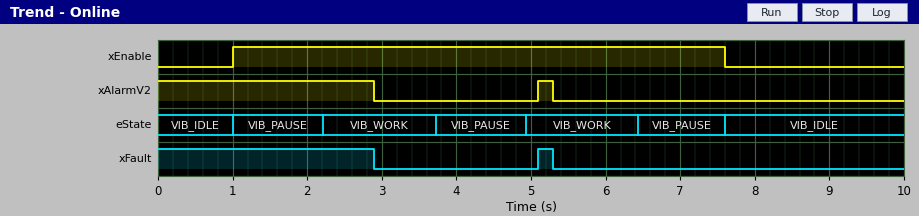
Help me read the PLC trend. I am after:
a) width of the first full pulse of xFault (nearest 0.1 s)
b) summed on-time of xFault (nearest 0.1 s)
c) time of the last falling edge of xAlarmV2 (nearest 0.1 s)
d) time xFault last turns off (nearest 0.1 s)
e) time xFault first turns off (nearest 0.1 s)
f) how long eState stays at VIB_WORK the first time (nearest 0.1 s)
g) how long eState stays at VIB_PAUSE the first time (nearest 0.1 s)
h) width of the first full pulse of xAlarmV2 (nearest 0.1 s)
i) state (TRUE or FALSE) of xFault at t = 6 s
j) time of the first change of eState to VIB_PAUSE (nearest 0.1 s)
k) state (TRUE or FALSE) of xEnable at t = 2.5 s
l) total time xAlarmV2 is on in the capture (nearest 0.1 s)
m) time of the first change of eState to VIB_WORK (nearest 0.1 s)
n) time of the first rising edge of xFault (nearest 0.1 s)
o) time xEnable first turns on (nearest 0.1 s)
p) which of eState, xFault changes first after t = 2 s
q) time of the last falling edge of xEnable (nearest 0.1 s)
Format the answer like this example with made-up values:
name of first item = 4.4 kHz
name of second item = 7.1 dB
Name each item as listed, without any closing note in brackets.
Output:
width of the first full pulse of xFault = 0.2 s
summed on-time of xFault = 3.1 s
time of the last falling edge of xAlarmV2 = 5.3 s
time xFault last turns off = 5.3 s
time xFault first turns off = 2.9 s
how long eState stays at VIB_WORK the first time = 1.5 s
how long eState stays at VIB_PAUSE the first time = 1.2 s
width of the first full pulse of xAlarmV2 = 0.2 s
state (TRUE or FALSE) of xFault at t = 6 s = FALSE
time of the first change of eState to VIB_PAUSE = 1.0 s
state (TRUE or FALSE) of xEnable at t = 2.5 s = TRUE
total time xAlarmV2 is on in the capture = 3.1 s
time of the first change of eState to VIB_WORK = 2.2 s
time of the first rising edge of xFault = 5.1 s
time xEnable first turns on = 1.0 s
which of eState, xFault changes first after t = 2 s = eState
time of the last falling edge of xEnable = 7.6 s
